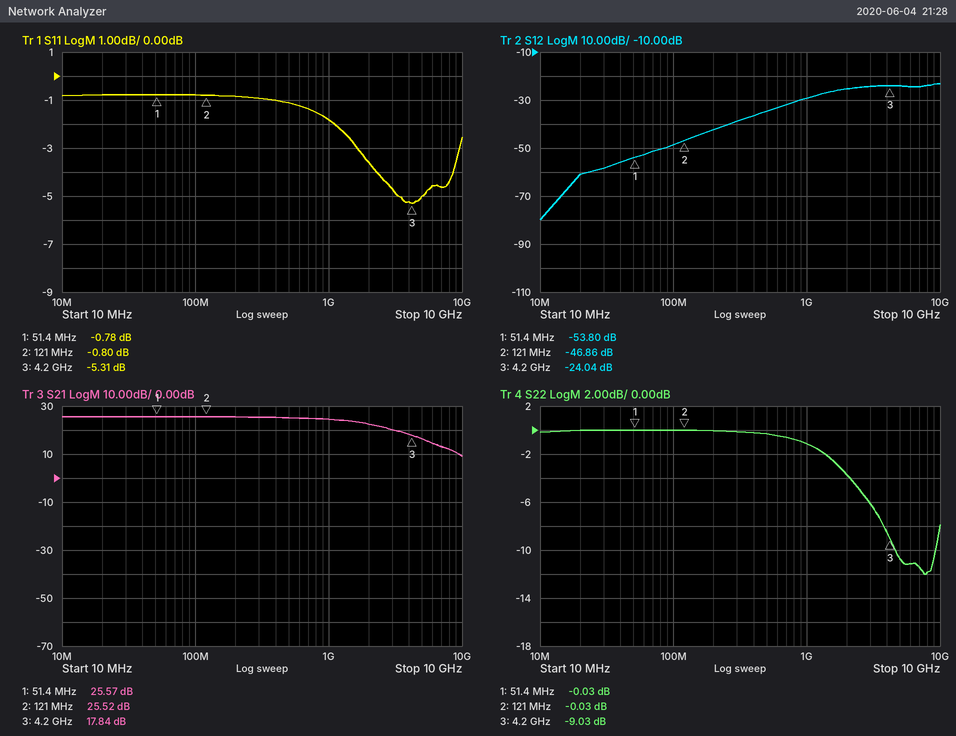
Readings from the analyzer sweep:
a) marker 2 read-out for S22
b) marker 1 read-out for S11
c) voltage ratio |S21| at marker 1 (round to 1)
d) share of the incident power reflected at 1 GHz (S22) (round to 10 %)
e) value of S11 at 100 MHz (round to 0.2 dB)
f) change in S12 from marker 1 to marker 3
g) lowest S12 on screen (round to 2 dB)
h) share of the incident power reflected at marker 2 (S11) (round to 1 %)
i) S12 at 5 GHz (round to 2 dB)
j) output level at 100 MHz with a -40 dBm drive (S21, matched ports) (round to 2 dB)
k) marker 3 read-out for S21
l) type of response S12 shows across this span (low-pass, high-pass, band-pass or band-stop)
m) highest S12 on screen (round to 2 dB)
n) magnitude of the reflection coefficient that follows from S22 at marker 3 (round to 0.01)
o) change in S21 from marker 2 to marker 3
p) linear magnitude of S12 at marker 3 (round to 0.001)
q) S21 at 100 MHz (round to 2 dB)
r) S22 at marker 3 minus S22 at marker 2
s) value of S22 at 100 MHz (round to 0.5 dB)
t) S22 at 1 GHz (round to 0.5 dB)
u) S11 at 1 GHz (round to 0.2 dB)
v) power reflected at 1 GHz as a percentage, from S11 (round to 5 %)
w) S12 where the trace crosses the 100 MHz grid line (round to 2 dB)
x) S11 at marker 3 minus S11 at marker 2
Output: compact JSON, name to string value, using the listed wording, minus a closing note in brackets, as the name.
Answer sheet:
{"marker 2 read-out for S22": "-0.03 dB", "marker 1 read-out for S11": "-0.78 dB", "voltage ratio |S21| at marker 1": "19", "share of the incident power reflected at 1 GHz (S22)": "80 %", "value of S11 at 100 MHz": "-0.8 dB", "change in S12 from marker 1 to marker 3": "29.76 dB", "lowest S12 on screen": "-80 dB", "share of the incident power reflected at marker 2 (S11)": "83 %", "S12 at 5 GHz": "-24 dB", "output level at 100 MHz with a -40 dBm drive (S21, matched ports)": "-14 dBm", "marker 3 read-out for S21": "17.84 dB", "type of response S12 shows across this span": "high-pass", "highest S12 on screen": "-24 dB", "magnitude of the reflection coefficient that follows from S22 at marker 3": "0.35", "change in S21 from marker 2 to marker 3": "-7.68 dB", "linear magnitude of S12 at marker 3": "0.063", "S21 at 100 MHz": "26 dB", "S22 at marker 3 minus S22 at marker 2": "-9.00 dB", "value of S22 at 100 MHz": "0.0 dB", "S22 at 1 GHz": "-1.0 dB", "S11 at 1 GHz": "-1.8 dB", "power reflected at 1 GHz as a percentage, from S11": "65 %", "S12 where the trace crosses the 100 MHz grid line": "-48 dB", "S11 at marker 3 minus S11 at marker 2": "-4.51 dB"}
